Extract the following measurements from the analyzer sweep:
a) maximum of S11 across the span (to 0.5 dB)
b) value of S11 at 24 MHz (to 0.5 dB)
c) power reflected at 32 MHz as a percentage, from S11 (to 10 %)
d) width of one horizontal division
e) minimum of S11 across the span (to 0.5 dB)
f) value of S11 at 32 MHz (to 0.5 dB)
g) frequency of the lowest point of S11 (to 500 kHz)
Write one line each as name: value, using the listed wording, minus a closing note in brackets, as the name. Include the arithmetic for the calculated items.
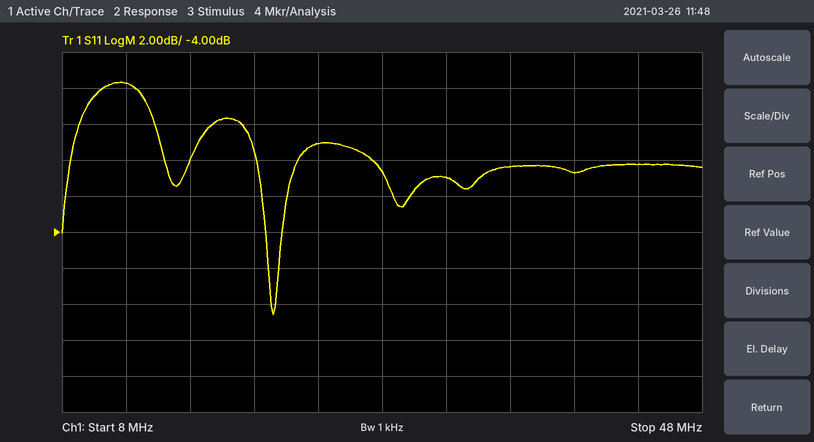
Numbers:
maximum of S11 across the span: 4.5 dB
value of S11 at 24 MHz: 1.0 dB
power reflected at 32 MHz as a percentage, from S11: 10^(-1/10) ≈ 79.4 %, so 80 % to the nearest 10 %
width of one horizontal division: 4 MHz
minimum of S11 across the span: -8.5 dB
value of S11 at 32 MHz: -1.0 dB
frequency of the lowest point of S11: 21.0 MHz
